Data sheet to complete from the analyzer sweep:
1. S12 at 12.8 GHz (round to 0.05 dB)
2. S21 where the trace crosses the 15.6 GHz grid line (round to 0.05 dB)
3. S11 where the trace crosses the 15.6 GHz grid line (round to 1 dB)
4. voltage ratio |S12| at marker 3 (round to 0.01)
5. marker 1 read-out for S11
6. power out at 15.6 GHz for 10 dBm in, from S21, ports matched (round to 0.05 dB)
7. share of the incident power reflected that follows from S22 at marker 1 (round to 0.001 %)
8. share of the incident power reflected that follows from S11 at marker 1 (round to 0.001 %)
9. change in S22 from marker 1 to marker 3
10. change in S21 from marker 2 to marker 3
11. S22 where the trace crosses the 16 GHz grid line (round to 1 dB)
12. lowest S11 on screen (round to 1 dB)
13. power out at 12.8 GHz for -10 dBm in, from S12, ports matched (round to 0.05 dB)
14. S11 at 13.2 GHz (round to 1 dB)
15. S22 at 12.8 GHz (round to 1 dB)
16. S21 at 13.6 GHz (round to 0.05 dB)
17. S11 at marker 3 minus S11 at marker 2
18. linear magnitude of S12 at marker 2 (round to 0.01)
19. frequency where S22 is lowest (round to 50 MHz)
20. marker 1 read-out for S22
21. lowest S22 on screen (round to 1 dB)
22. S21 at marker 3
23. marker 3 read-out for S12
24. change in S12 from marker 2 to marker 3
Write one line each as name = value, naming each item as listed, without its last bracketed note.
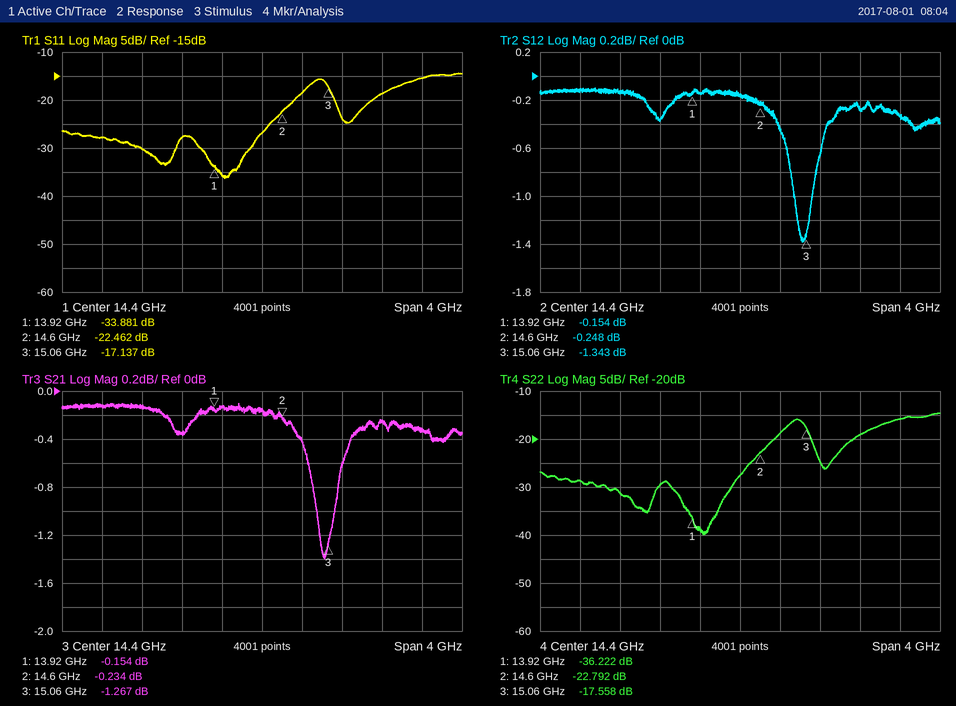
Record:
S12 at 12.8 GHz = -0.10 dB
S21 where the trace crosses the 15.6 GHz grid line = -0.25 dB
S11 where the trace crosses the 15.6 GHz grid line = -19 dB
voltage ratio |S12| at marker 3 = 0.86
marker 1 read-out for S11 = -33.881 dB
power out at 15.6 GHz for 10 dBm in, from S21, ports matched = 9.75 dBm
share of the incident power reflected that follows from S22 at marker 1 = 0.024 %
share of the incident power reflected that follows from S11 at marker 1 = 0.041 %
change in S22 from marker 1 to marker 3 = 18.664 dB
change in S21 from marker 2 to marker 3 = -1.033 dB
S22 where the trace crosses the 16 GHz grid line = -16 dB
lowest S11 on screen = -36 dB
power out at 12.8 GHz for -10 dBm in, from S12, ports matched = -10.10 dBm
S11 at 13.2 GHz = -30 dB
S22 at 12.8 GHz = -29 dB
S21 at 13.6 GHz = -0.35 dB
S11 at marker 3 minus S11 at marker 2 = 5.325 dB
linear magnitude of S12 at marker 2 = 0.97
frequency where S22 is lowest = 14.05 GHz
marker 1 read-out for S22 = -36.222 dB
lowest S22 on screen = -40 dB
S21 at marker 3 = -1.267 dB
marker 3 read-out for S12 = -1.343 dB
change in S12 from marker 2 to marker 3 = -1.095 dB
